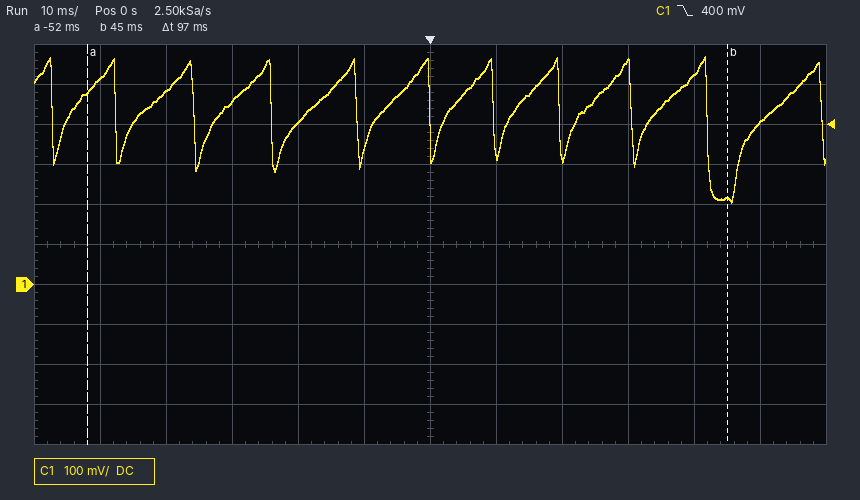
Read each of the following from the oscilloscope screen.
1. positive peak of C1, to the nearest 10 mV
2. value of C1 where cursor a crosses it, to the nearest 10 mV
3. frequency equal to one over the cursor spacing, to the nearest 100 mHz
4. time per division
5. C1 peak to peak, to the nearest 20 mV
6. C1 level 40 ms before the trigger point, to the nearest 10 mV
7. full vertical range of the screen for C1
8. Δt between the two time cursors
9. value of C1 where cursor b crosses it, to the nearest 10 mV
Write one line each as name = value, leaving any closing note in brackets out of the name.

positive peak of C1, to the nearest 10 mV = 570 mV
value of C1 where cursor a crosses it, to the nearest 10 mV = 480 mV
frequency equal to one over the cursor spacing, to the nearest 100 mHz = 10.3 Hz
time per division = 10 ms
C1 peak to peak, to the nearest 20 mV = 360 mV
C1 level 40 ms before the trigger point, to the nearest 10 mV = 480 mV
full vertical range of the screen for C1 = 1 V
Δt between the two time cursors = 97 ms
value of C1 where cursor b crosses it, to the nearest 10 mV = 210 mV
